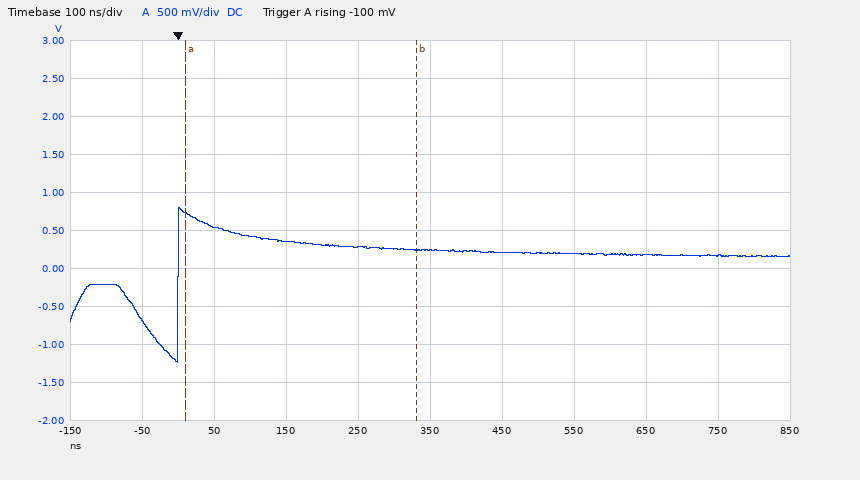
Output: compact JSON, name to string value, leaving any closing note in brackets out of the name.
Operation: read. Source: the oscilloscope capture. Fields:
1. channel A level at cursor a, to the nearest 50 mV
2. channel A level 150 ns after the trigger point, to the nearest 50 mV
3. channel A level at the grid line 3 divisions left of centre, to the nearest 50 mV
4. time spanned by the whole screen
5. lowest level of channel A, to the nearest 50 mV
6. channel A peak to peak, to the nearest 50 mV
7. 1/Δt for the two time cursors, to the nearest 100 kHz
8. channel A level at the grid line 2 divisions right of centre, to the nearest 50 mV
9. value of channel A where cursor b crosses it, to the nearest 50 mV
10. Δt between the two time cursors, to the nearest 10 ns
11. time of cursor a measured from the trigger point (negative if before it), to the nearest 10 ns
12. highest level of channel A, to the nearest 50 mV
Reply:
{"channel A level at cursor a, to the nearest 50 mV": "750 mV", "channel A level 150 ns after the trigger point, to the nearest 50 mV": "350 mV", "channel A level at the grid line 3 divisions left of centre, to the nearest 50 mV": "550 mV", "time spanned by the whole screen": "1 µs", "lowest level of channel A, to the nearest 50 mV": "-1.25 V", "channel A peak to peak, to the nearest 50 mV": "2.05 V", "1/Δt for the two time cursors, to the nearest 100 kHz": "3.1 MHz", "channel A level at the grid line 2 divisions right of centre, to the nearest 50 mV": "200 mV", "value of channel A where cursor b crosses it, to the nearest 50 mV": "250 mV", "Δt between the two time cursors, to the nearest 10 ns": "320 ns", "time of cursor a measured from the trigger point (negative if before it), to the nearest 10 ns": "+10 ns", "highest level of channel A, to the nearest 50 mV": "800 mV"}
